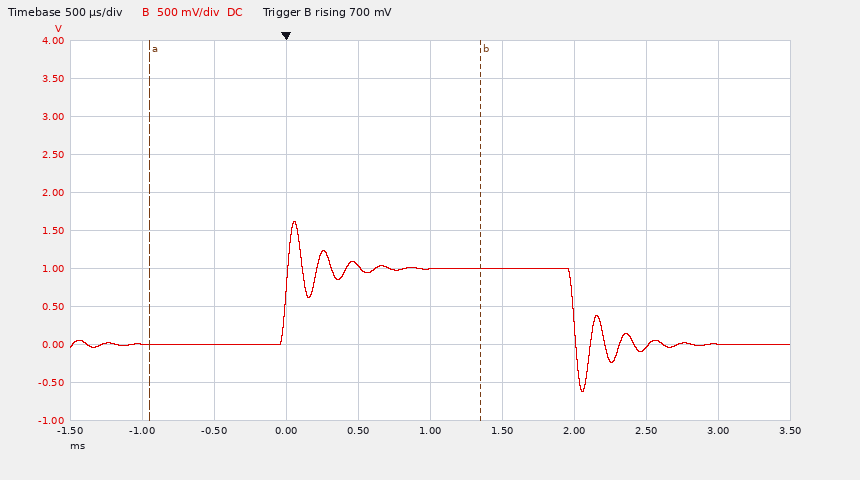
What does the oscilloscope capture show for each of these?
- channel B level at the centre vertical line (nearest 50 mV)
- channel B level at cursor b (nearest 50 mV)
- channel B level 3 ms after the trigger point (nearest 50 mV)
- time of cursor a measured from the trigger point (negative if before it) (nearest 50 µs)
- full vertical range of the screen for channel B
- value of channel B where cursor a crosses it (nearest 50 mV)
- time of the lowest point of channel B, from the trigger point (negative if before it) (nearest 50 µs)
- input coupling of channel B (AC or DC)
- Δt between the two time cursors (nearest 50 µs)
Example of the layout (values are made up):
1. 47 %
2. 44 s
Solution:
1. 1.00 V
2. 1.00 V
3. 0 mV
4. -950 µs
5. 5 V
6. 0 mV
7. +2.05 ms
8. DC
9. 2.30 ms
